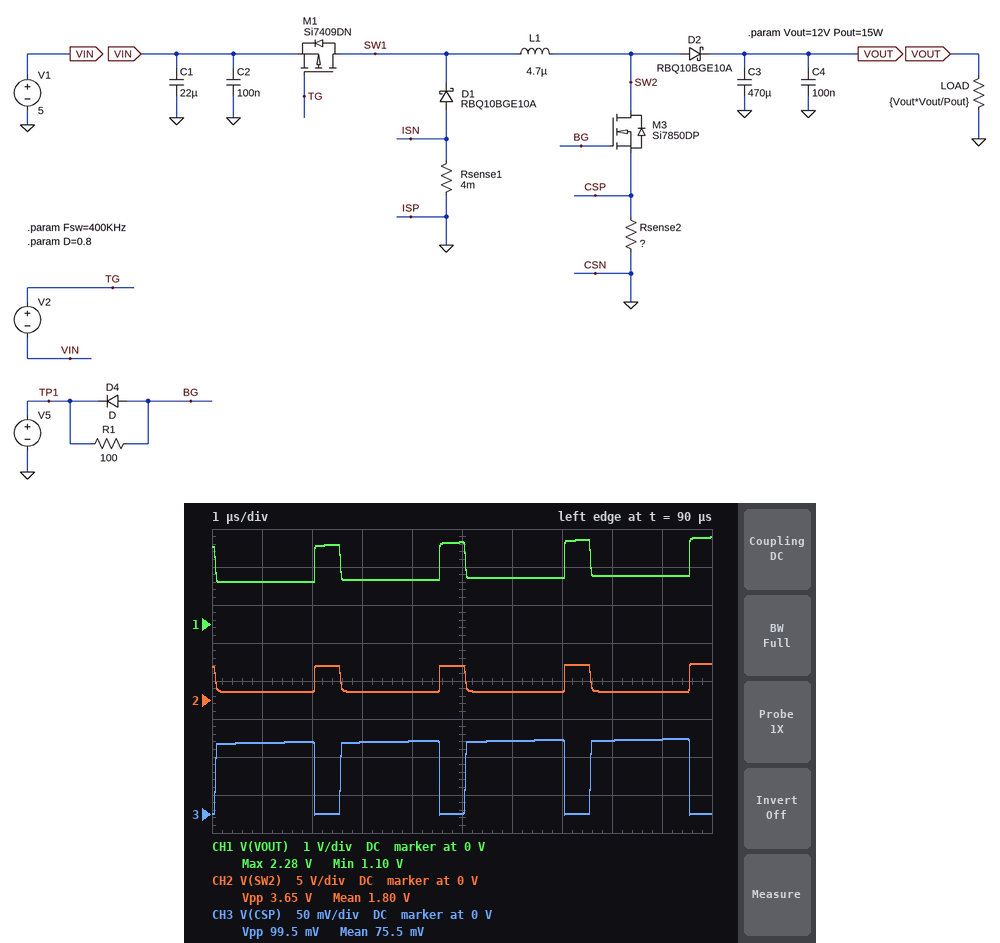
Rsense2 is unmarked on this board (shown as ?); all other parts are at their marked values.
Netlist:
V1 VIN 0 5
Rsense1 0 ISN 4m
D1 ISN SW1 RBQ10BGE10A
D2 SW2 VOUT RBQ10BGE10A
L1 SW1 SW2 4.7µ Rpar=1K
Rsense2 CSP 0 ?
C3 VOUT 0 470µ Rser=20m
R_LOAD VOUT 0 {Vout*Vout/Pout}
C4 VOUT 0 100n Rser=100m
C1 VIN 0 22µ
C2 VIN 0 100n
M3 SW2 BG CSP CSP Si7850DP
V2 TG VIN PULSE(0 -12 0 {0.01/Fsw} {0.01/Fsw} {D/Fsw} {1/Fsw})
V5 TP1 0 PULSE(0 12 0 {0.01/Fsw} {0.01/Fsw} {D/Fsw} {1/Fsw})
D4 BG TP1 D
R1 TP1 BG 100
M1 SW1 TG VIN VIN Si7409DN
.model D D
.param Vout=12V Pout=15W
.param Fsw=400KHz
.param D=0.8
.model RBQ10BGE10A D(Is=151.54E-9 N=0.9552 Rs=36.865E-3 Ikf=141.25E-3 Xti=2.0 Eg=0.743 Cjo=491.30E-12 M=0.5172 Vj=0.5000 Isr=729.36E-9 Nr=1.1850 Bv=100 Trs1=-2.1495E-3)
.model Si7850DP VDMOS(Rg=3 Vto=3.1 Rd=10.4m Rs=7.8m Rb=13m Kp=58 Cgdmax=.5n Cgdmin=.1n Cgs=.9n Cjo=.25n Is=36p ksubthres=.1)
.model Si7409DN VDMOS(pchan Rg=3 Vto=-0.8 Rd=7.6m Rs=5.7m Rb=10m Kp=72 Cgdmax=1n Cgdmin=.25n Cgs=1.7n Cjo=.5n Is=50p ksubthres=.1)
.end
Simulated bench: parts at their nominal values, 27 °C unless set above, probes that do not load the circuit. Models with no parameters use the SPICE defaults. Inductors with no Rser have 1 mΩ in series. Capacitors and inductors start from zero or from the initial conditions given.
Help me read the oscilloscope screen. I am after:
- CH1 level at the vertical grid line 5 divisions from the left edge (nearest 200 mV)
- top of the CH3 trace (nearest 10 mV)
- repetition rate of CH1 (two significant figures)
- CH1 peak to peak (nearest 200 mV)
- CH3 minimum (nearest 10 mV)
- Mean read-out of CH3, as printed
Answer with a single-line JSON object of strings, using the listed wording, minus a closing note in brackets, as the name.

{"CH1 level at the vertical grid line 5 divisions from the left edge": "2.2 V", "top of the CH3 trace": "100 mV", "repetition rate of CH1": "400 kHz", "CH1 peak to peak": "1.2 V", "CH3 minimum": "0 V", "Mean read-out of CH3, as printed": "75.5 mV"}
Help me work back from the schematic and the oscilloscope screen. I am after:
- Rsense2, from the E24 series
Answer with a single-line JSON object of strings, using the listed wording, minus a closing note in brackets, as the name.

{"Rsense2, from the E24 series": "2 mΩ"}
